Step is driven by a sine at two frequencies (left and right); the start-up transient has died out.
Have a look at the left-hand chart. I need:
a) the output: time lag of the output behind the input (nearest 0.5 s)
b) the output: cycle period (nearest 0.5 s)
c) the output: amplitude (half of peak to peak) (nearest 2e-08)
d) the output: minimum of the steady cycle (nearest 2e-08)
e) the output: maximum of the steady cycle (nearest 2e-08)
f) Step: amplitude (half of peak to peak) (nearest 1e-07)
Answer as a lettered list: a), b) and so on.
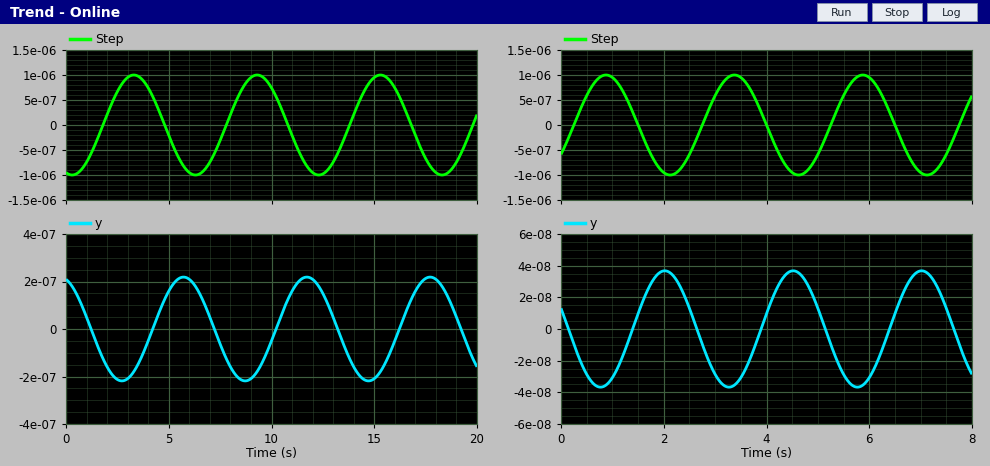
a) 2.5 s
b) 6.0 s
c) 0.00000022
d) -0.00000022
e) 0.00000022
f) 0.0000010
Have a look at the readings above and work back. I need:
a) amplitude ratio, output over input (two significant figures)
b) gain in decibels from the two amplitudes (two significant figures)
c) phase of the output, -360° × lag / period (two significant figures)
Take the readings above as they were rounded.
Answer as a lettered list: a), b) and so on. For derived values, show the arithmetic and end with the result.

a) 2.2e-07 / 1e-06 = 0.22
b) 20 log10(2.2e-07 / 1e-06) = -13 dB
c) -360 × 2.5 / 6 = -150°
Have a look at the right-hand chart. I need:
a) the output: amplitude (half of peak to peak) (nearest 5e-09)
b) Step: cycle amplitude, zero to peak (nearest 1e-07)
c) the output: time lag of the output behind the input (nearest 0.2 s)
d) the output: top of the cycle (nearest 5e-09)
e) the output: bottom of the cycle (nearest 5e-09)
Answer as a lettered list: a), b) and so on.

a) 0.000000035
b) 0.0000010
c) 1.2 s
d) 0.000000035
e) -0.000000035
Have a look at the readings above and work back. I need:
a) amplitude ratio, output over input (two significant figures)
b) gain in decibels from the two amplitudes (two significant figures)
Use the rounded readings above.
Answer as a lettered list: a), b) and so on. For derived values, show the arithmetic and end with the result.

a) 3.5e-08 / 1e-06 = 0.035
b) 20 log10(3.5e-08 / 1e-06) = -29 dB
